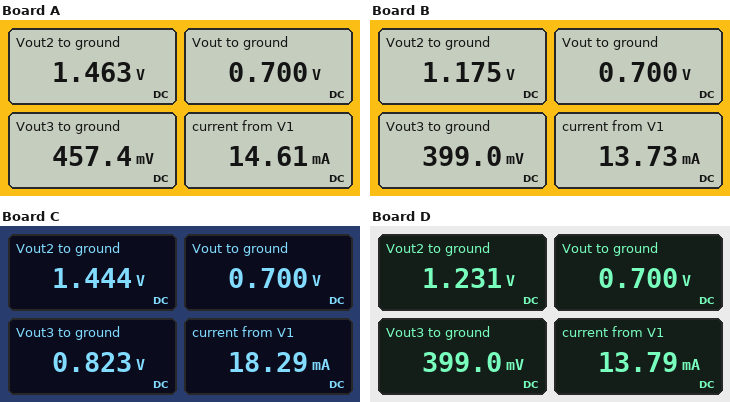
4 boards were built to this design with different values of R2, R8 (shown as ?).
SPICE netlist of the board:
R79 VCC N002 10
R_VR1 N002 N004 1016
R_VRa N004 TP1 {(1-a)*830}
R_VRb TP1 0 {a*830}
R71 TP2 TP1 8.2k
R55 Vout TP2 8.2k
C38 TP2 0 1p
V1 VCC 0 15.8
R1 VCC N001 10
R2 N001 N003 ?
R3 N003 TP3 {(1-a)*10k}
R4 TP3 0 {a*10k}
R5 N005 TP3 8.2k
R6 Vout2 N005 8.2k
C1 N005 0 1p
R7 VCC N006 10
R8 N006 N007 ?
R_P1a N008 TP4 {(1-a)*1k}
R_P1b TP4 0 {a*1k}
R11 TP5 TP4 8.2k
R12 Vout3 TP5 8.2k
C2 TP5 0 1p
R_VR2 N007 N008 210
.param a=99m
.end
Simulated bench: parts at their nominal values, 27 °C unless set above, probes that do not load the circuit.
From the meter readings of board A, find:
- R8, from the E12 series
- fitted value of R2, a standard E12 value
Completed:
2.2 kΩ
680 Ω
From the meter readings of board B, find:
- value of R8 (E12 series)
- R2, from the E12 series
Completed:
2.7 kΩ
3.3 kΩ
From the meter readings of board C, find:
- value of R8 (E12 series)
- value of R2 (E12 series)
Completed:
680 Ω
820 Ω
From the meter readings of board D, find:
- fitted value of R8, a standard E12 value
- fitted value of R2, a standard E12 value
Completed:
2.7 kΩ
2.7 kΩ
